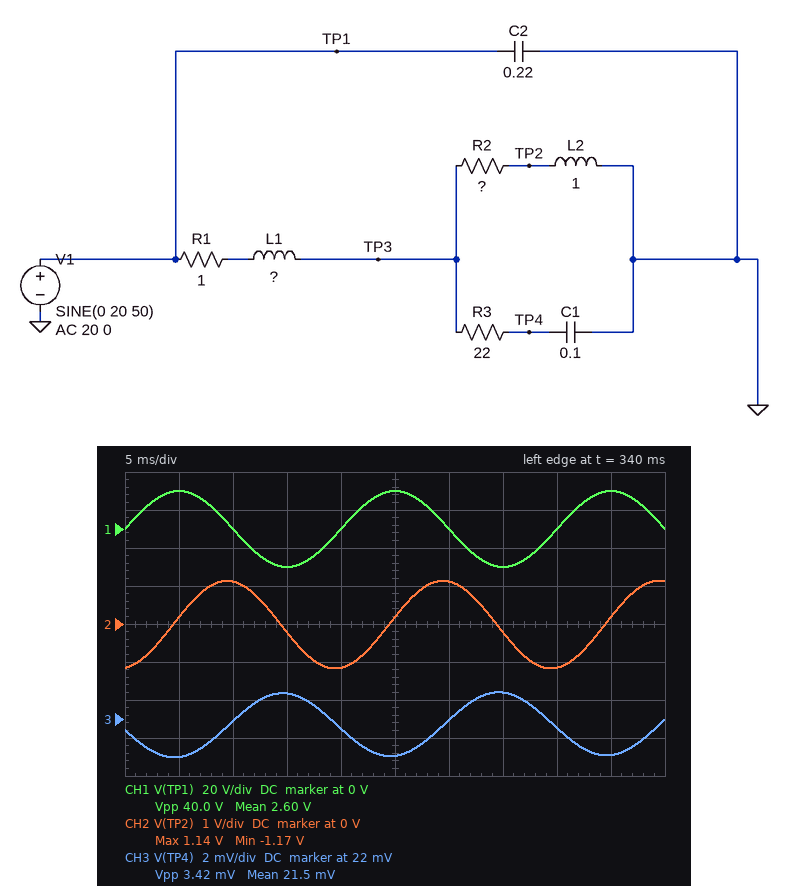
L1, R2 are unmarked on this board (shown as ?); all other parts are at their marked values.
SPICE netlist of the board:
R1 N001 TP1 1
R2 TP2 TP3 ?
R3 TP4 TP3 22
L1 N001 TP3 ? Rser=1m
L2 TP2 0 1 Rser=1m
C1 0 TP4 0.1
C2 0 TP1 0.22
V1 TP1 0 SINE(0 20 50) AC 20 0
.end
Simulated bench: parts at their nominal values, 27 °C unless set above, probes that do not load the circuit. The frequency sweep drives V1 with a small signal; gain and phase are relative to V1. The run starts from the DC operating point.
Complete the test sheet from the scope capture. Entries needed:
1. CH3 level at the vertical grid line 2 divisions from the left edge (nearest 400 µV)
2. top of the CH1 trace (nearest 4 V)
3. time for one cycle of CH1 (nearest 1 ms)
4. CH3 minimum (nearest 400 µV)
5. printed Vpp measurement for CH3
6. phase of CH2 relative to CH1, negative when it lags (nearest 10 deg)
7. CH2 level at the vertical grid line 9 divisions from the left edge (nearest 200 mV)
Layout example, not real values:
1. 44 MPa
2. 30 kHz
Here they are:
1. 22.0 mV
2. 20 V
3. 20 ms
4. 20.0 mV
5. 3.42 mV
6. -80 deg
7. 200 mV
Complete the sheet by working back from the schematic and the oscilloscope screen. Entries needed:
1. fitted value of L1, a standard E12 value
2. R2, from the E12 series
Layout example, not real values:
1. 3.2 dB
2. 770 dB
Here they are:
1. 1.2 H
2. 15 Ω
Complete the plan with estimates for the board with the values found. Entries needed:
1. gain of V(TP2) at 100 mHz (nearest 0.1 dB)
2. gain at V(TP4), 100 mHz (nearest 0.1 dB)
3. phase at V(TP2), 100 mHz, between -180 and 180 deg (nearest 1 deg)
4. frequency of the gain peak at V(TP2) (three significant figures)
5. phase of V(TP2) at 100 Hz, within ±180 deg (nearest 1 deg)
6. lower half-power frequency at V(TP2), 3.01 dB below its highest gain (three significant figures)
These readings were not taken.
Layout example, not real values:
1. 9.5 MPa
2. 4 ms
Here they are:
1. -28.3 dB
2. -5.4 dB
3. 83 deg
4. 2.75 Hz
5. -85 deg
6. 785 mHz
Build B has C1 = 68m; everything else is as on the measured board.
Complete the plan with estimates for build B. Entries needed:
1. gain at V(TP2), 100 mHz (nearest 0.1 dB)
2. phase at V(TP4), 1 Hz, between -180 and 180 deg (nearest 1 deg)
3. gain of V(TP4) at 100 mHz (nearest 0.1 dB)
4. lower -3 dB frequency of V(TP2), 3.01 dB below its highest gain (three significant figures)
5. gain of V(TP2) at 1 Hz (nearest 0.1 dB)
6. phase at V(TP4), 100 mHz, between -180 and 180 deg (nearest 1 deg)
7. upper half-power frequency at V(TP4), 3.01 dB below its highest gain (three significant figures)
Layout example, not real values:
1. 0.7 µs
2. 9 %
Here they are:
1. -28.2 dB
2. -115 deg
3. -3.4 dB
4. 780 mHz
5. -11.5 dB
6. -48 deg
7. 104 mHz
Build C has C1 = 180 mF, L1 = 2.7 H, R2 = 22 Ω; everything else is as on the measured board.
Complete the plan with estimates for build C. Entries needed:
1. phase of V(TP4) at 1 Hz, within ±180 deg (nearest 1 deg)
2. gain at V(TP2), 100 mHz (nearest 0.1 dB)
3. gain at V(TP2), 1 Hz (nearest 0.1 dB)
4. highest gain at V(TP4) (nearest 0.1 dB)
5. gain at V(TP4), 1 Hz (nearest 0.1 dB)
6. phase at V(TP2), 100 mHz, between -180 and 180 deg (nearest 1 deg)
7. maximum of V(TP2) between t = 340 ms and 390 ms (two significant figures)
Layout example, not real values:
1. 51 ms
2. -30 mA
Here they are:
1. -137 deg
2. -31.5 dB
3. -17.0 dB
4. -0.4 dB
5. -33.7 dB
6. 80 deg
7. 500 mV
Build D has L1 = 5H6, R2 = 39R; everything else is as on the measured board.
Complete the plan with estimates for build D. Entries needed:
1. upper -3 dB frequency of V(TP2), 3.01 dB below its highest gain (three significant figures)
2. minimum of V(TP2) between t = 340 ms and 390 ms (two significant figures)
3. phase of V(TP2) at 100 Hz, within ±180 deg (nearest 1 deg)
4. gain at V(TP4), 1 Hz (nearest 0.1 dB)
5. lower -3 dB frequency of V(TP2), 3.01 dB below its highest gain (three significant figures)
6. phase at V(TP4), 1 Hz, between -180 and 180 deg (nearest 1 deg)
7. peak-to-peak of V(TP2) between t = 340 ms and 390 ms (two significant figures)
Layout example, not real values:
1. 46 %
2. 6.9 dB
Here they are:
1. 10.6 Hz
2. -250 mV
3. -84 deg
4. -31.5 dB
5. 345 mHz
6. -152 deg
7. 490 mV
